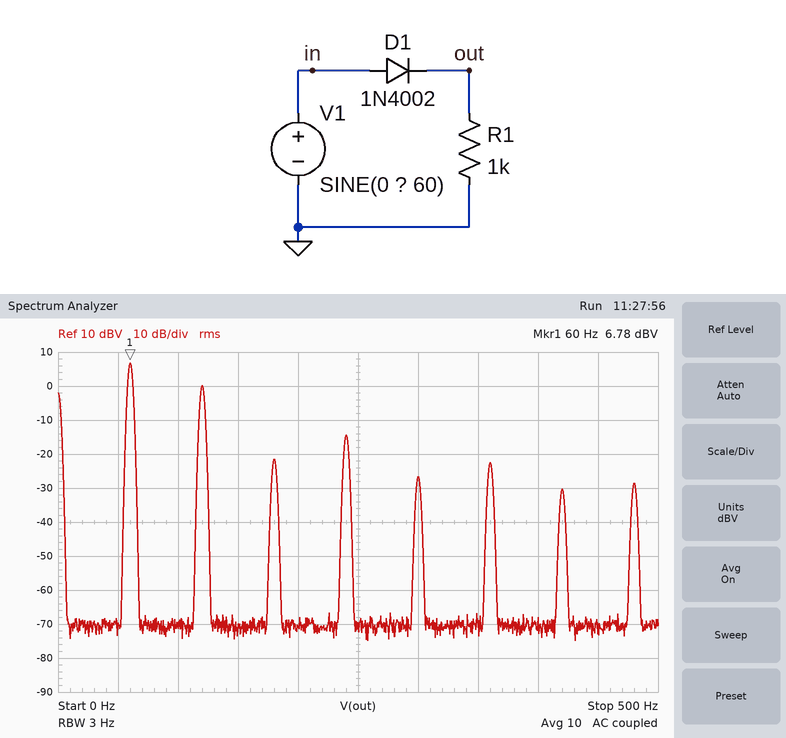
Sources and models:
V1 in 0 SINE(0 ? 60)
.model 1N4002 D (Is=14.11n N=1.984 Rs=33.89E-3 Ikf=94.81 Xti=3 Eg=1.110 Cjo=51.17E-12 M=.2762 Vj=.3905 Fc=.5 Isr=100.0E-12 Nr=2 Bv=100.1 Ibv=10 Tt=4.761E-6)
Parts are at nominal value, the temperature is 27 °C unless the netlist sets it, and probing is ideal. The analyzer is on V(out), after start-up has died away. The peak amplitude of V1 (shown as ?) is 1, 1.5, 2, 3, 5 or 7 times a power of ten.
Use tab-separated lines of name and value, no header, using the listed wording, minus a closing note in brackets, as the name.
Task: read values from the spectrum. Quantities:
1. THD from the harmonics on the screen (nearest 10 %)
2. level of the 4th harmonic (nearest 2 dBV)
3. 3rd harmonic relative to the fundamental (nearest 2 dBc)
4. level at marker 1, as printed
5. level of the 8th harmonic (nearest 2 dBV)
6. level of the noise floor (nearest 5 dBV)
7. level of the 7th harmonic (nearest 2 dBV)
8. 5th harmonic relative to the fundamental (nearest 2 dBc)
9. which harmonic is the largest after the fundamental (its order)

THD from the harmonics on the screen	50 %
level of the 4th harmonic	-14 dBV
3rd harmonic relative to the fundamental	-28 dBc
level at marker 1, as printed	6.78 dBV
level of the 8th harmonic	-28 dBV
level of the noise floor	-70 dBV
level of the 7th harmonic	-30 dBV
5th harmonic relative to the fundamental	-34 dBc
which harmonic is the largest after the fundamental	2
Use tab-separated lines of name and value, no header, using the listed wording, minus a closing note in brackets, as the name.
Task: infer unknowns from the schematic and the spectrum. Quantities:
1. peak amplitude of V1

peak amplitude of V1	7 V
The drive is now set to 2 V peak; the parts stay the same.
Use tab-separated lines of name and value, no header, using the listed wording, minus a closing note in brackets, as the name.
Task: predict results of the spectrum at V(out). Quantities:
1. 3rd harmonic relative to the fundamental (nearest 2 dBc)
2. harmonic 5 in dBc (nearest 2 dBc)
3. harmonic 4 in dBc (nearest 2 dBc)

3rd harmonic relative to the fundamental	-18 dBc
harmonic 5 in dBc	-24 dBc
harmonic 4 in dBc	-24 dBc
